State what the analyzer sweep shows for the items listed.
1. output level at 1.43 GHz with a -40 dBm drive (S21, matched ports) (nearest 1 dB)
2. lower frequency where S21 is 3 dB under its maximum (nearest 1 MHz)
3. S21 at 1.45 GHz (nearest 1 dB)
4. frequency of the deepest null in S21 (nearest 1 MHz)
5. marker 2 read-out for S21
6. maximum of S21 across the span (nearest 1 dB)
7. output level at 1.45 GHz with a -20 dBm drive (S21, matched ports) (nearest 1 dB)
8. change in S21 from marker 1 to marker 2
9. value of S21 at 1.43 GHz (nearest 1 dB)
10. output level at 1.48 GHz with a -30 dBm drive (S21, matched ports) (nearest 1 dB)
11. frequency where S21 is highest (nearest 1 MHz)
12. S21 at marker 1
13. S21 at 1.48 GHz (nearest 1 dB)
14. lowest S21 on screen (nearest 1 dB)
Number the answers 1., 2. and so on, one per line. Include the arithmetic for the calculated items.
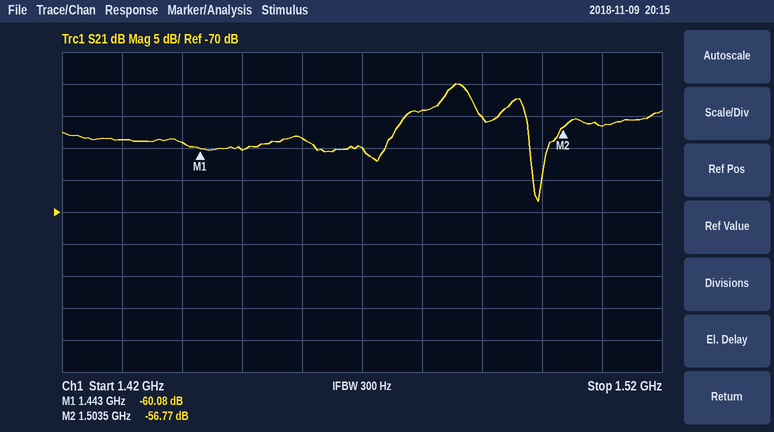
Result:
1. -40 dBm + (-59 dB) = -99 dBm
2. 1.483 GHz
3. -60 dB
4. 1.499 GHz
5. -56.77 dB
6. -50 dB
7. -20 dBm + (-60 dB) = -80 dBm
8. -56.77 − (-60.08) = 3.31 dB
9. -59 dB
10. -30 dBm + (-54 dB) = -84 dBm
11. 1.486 GHz
12. -60.08 dB
13. -54 dB
14. -68 dB
